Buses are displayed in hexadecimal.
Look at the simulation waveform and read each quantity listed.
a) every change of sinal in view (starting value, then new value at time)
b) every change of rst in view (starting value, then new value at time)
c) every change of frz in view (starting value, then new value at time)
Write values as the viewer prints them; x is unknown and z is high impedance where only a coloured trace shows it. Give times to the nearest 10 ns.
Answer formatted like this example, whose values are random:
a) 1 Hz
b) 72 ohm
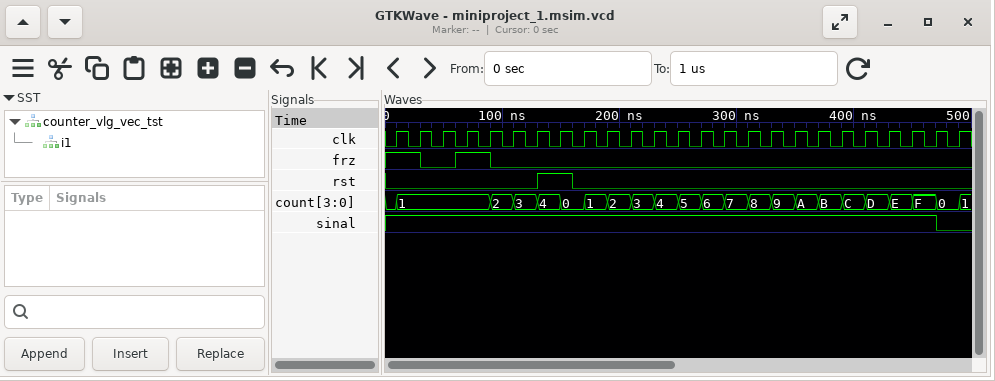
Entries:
a) 1, 0 at 470 ns
b) 0, 1 at 130 ns, 0 at 160 ns
c) 1, 0 at 30 ns, 1 at 60 ns, 0 at 90 ns
